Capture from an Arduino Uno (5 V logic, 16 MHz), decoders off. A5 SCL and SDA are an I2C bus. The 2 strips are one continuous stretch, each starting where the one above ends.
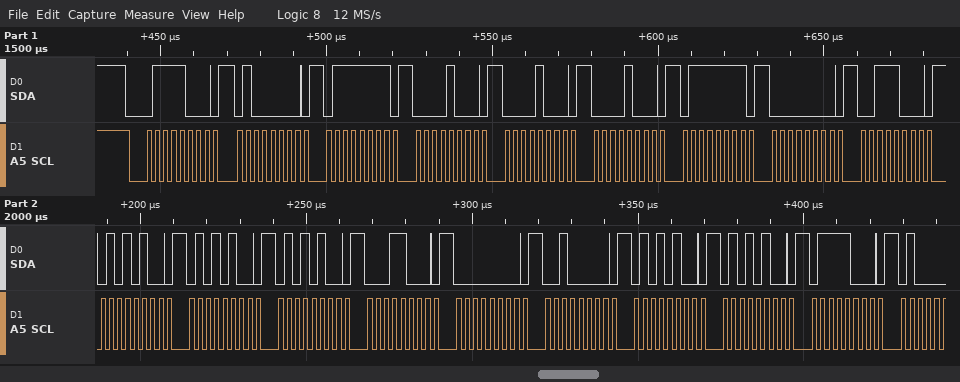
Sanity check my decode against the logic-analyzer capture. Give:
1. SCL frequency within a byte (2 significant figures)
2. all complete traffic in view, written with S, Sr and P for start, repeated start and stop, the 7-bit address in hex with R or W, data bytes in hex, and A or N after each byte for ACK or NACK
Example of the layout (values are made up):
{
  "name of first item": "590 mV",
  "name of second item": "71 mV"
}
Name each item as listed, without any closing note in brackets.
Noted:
{
  "SCL frequency within a byte": "400 kHz",
  "all complete traffic in view, written with S, Sr and P for start, repeated start and stop, the 7-bit address in hex with R or W, data bytes in hex, and A or N after each byte for ACK or NACK": "S 3CW A 40 A 7F A 08 A 08 A 08 A 7F A 00 A 38 A 54 A 54 A 54 A 18 A 00 A 20 A 54 A 54 A 78 A"
}
